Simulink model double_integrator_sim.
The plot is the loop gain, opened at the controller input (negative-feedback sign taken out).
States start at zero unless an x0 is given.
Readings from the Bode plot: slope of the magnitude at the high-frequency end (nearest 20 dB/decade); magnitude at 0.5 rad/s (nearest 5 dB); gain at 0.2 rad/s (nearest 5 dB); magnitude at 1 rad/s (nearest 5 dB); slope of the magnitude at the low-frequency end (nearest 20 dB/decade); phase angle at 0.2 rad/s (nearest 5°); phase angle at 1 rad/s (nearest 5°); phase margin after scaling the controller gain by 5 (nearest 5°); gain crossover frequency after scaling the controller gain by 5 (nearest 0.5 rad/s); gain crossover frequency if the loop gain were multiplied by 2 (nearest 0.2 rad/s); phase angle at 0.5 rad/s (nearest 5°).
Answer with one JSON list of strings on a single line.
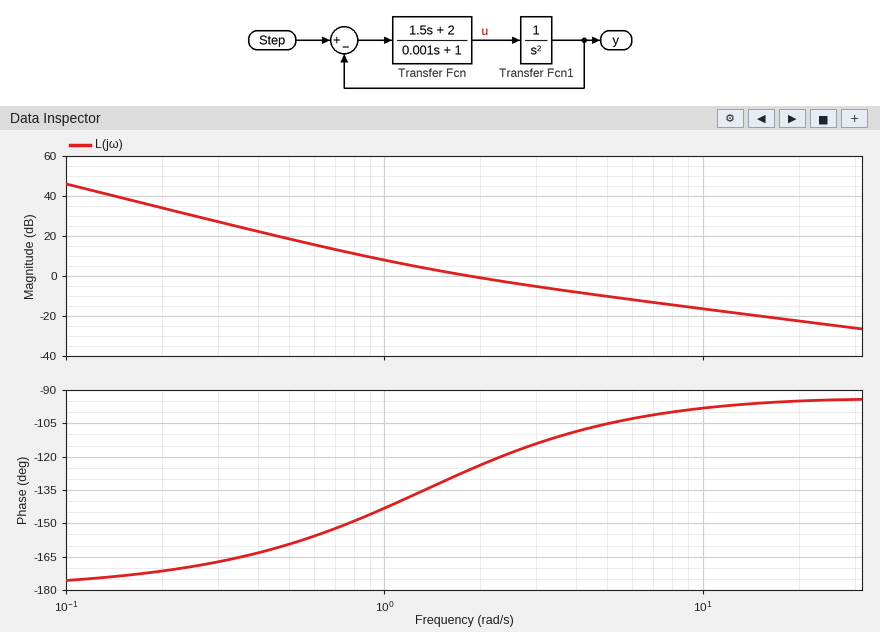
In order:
["-20 dB/decade", "20 dB", "35 dB", "10 dB", "-40 dB/decade", "-170°", "-145°", "80°", "7.5 rad/s", "3.2 rad/s", "-160°"]
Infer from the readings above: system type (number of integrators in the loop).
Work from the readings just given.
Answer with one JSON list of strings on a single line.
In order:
["2"]
